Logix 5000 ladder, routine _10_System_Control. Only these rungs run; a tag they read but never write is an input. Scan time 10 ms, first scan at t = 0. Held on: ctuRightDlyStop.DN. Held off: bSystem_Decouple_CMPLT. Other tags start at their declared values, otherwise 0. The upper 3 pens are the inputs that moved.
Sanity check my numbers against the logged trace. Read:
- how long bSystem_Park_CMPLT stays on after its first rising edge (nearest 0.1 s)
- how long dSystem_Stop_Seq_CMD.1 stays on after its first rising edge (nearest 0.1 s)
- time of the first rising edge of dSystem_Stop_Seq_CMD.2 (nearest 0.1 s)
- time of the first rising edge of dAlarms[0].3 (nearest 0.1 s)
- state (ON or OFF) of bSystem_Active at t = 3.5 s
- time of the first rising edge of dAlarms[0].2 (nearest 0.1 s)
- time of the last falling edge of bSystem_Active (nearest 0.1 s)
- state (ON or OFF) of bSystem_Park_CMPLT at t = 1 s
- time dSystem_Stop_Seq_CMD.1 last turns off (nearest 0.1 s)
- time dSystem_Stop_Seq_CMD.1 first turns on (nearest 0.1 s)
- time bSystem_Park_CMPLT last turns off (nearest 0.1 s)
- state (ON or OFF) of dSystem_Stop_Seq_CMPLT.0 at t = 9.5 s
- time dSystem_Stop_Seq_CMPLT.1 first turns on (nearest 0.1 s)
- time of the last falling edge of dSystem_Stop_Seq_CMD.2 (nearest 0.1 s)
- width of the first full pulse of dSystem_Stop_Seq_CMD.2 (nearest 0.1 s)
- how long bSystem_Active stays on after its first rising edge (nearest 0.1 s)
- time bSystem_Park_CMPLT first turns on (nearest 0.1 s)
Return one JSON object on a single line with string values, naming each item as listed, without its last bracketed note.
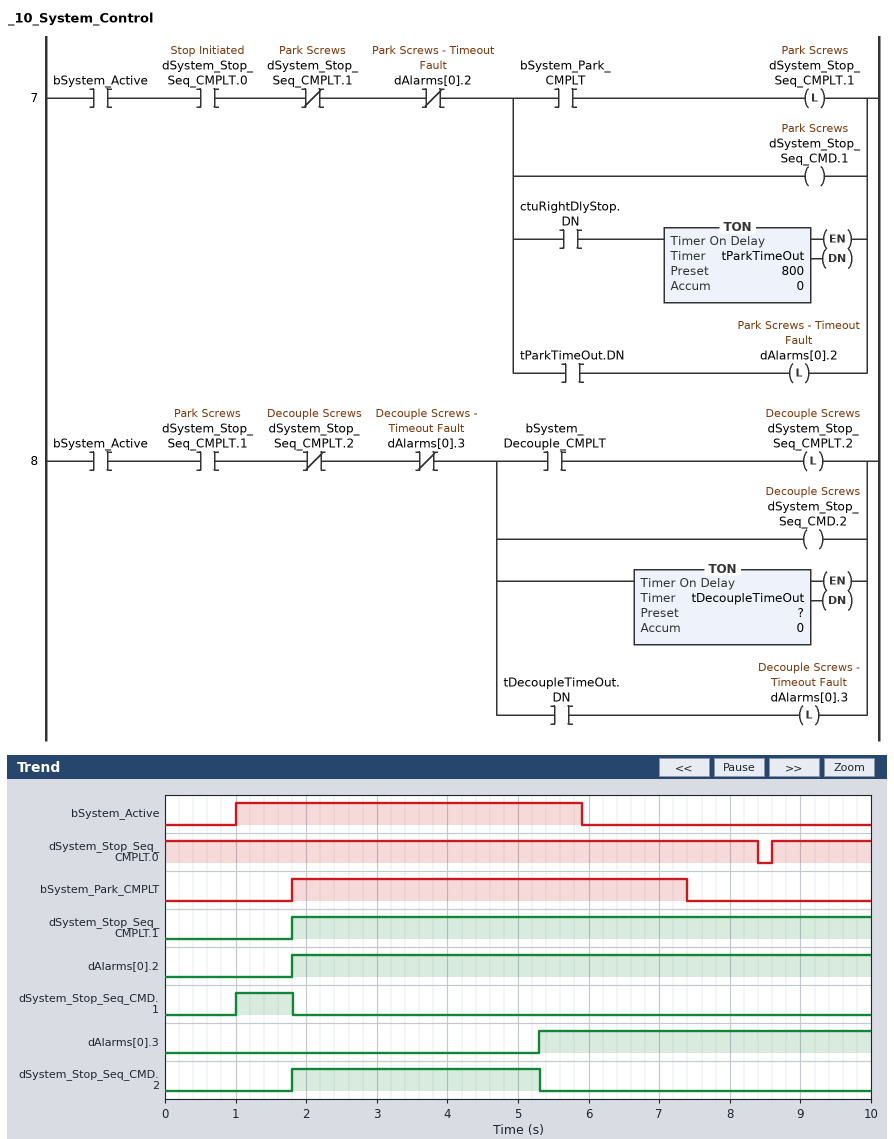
{"how long bSystem_Park_CMPLT stays on after its first rising edge": "5.6 s", "how long dSystem_Stop_Seq_CMD.1 stays on after its first rising edge": "0.8 s", "time of the first rising edge of dSystem_Stop_Seq_CMD.2": "1.8 s", "time of the first rising edge of dAlarms[0].3": "5.3 s", "state (ON or OFF) of bSystem_Active at t = 3.5 s": "ON", "time of the first rising edge of dAlarms[0].2": "1.8 s", "time of the last falling edge of bSystem_Active": "5.9 s", "state (ON or OFF) of bSystem_Park_CMPLT at t = 1 s": "OFF", "time dSystem_Stop_Seq_CMD.1 last turns off": "1.8 s", "time dSystem_Stop_Seq_CMD.1 first turns on": "1.0 s", "time bSystem_Park_CMPLT last turns off": "7.4 s", "state (ON or OFF) of dSystem_Stop_Seq_CMPLT.0 at t = 9.5 s": "ON", "time dSystem_Stop_Seq_CMPLT.1 first turns on": "1.8 s", "time of the last falling edge of dSystem_Stop_Seq_CMD.2": "5.3 s", "width of the first full pulse of dSystem_Stop_Seq_CMD.2": "3.5 s", "how long bSystem_Active stays on after its first rising edge": "4.9 s", "time bSystem_Park_CMPLT first turns on": "1.8 s"}
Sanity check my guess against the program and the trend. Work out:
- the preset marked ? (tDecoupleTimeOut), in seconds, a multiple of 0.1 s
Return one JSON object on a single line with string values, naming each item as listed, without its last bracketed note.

{"the preset marked ? (tDecoupleTimeOut), in seconds, a multiple of 0.1 s": "3.5 s"}
